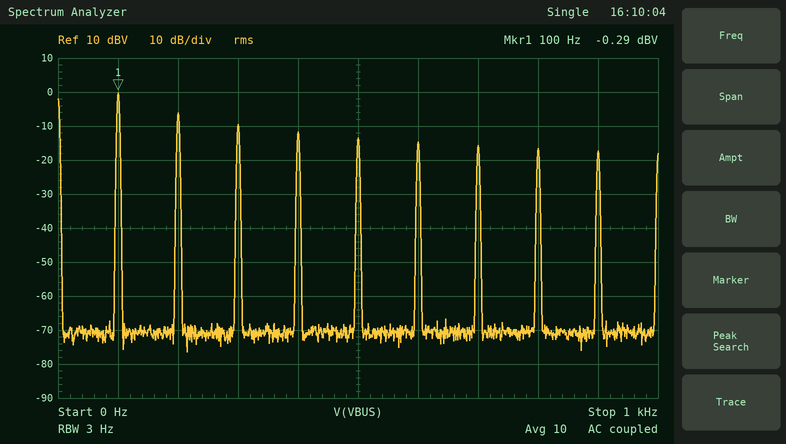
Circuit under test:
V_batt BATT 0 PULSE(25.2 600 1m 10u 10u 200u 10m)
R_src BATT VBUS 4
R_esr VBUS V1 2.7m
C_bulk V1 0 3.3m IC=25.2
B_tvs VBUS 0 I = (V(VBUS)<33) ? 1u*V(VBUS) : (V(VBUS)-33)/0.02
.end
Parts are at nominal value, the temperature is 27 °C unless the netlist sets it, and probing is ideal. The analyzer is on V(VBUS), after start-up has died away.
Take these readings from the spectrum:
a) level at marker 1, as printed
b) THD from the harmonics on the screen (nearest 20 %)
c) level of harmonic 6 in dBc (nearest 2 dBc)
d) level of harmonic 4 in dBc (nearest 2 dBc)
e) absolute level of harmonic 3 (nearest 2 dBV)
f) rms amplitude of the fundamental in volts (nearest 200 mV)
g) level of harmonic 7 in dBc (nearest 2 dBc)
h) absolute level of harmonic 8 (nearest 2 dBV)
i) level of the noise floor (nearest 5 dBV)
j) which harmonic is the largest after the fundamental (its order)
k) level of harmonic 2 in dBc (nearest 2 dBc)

-0.29 dBV
80 %
-14 dBc
-12 dBc
-10 dBV
1.0 V
-16 dBc
-16 dBV
-70 dBV
2
-6 dBc
